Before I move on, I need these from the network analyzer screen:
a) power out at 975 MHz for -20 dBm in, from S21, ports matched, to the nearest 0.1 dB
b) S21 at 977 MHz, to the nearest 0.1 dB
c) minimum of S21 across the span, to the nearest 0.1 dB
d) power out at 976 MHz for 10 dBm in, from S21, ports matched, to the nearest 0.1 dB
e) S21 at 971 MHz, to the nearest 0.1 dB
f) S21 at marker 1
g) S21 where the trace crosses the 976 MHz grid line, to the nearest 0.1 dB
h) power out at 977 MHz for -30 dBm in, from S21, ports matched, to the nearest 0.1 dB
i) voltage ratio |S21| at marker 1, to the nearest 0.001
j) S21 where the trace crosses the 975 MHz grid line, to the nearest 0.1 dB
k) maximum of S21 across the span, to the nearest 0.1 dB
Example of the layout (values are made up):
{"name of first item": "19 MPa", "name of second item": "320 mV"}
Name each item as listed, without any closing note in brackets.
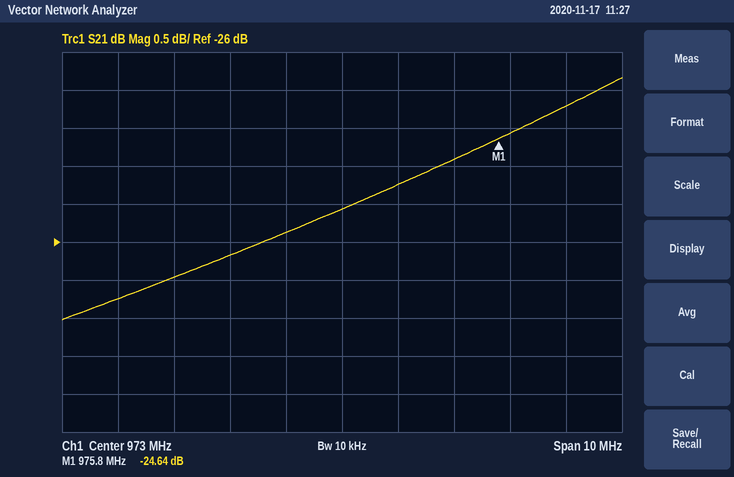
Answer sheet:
{"power out at 975 MHz for -20 dBm in, from S21, ports matched, to the nearest 0.1 dB": "-44.9 dBm", "S21 at 977 MHz, to the nearest 0.1 dB": "-24.2 dB", "minimum of S21 across the span, to the nearest 0.1 dB": "-27.0 dB", "power out at 976 MHz for 10 dBm in, from S21, ports matched, to the nearest 0.1 dB": "-14.6 dBm", "S21 at 971 MHz, to the nearest 0.1 dB": "-26.2 dB", "S21 at marker 1": "-24.64 dB", "S21 where the trace crosses the 976 MHz grid line, to the nearest 0.1 dB": "-24.6 dB", "power out at 977 MHz for -30 dBm in, from S21, ports matched, to the nearest 0.1 dB": "-54.2 dBm", "voltage ratio |S21| at marker 1, to the nearest 0.001": "0.059", "S21 where the trace crosses the 975 MHz grid line, to the nearest 0.1 dB": "-24.9 dB", "maximum of S21 across the span, to the nearest 0.1 dB": "-23.8 dB"}
